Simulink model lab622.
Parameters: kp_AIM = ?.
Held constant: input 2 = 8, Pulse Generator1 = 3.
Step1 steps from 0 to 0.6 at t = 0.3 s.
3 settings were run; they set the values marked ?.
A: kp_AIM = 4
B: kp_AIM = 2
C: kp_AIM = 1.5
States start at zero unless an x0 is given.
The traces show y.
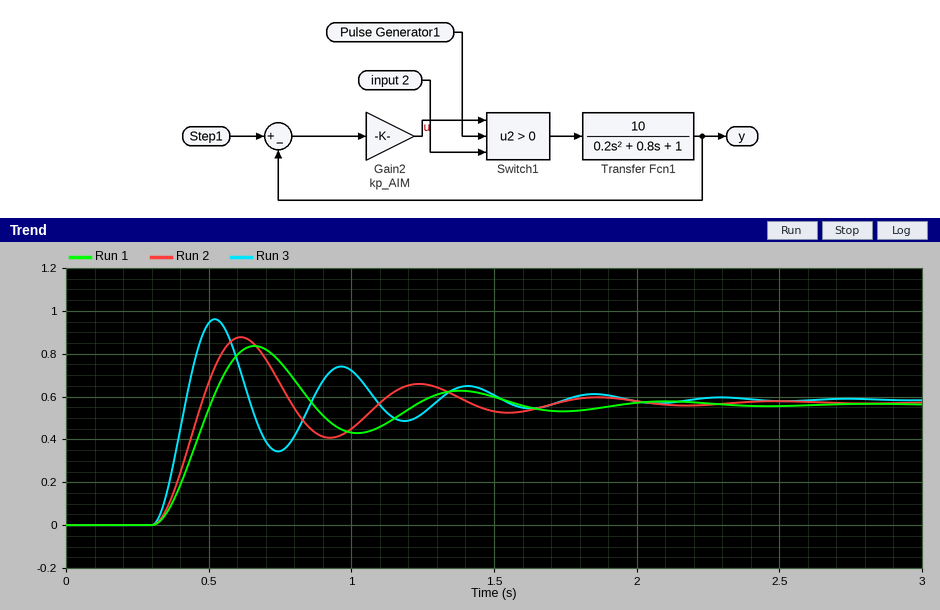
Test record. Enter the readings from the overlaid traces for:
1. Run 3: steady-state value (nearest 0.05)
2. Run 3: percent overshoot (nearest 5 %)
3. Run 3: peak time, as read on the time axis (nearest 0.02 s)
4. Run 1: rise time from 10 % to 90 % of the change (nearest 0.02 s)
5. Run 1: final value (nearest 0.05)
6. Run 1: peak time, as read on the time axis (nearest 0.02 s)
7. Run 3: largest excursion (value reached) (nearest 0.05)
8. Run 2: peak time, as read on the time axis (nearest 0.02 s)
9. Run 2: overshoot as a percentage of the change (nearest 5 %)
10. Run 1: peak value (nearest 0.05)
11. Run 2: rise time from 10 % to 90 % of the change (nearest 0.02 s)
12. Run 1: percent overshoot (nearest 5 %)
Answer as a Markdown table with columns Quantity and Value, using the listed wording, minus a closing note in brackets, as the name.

| Quantity | Value |
|---|---|
| Run 3: steady-state value | 0.60 |
| Run 3: percent overshoot | 65 % |
| Run 3: peak time, as read on the time axis | 0.52 s |
| Run 1: rise time from 10 % to 90 % of the change | 0.14 s |
| Run 1: final value | 0.55 |
| Run 1: peak time, as read on the time axis | 0.66 s |
| Run 3: largest excursion (value reached) | 0.95 |
| Run 2: peak time, as read on the time axis | 0.62 s |
| Run 2: overshoot as a percentage of the change | 55 % |
| Run 1: peak value | 0.85 |
| Run 2: rise time from 10 % to 90 % of the change | 0.12 s |
| Run 1: percent overshoot | 50 % |
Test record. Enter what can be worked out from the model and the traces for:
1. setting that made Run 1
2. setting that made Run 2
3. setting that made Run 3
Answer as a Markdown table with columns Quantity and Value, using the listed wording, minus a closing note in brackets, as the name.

| Quantity | Value |
|---|---|
| setting that made Run 1 | C |
| setting that made Run 2 | B |
| setting that made Run 3 | A |
